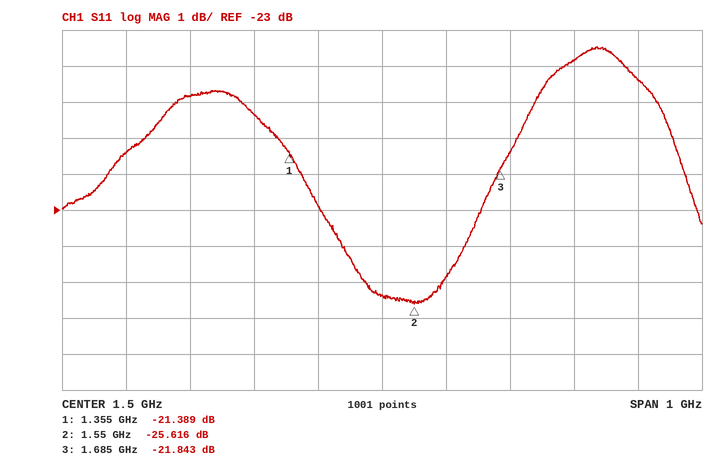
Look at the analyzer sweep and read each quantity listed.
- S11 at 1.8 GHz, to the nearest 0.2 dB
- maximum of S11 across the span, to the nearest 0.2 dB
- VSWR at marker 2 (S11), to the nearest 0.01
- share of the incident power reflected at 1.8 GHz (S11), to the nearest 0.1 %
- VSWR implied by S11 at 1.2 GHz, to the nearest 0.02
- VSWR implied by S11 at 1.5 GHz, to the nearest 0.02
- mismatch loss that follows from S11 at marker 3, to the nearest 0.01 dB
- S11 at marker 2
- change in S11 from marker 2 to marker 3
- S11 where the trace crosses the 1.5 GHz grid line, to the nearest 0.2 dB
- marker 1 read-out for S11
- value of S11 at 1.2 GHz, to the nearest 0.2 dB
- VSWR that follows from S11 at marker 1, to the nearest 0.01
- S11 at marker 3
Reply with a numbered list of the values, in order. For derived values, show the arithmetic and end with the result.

1. -18.8 dB
2. -18.4 dB
3. (1 + 0.0524)/(1 − 0.0524) ≈ 1.11
4. 10^(-18.8/10) ≈ 1.3 %
5. |Γ| = 10^(-19.8/20) = 0.1023; VSWR = (1 + 0.1023)/(1 − 0.1023) ≈ 1.23, so 1.22 to the nearest 0.02
6. |Γ| = 10^(-25.4/20) = 0.0537; VSWR = (1 + 0.0537)/(1 − 0.0537) ≈ 1.11, so 1.12 to the nearest 0.02
7. −10 log10(1 − 10^(-21.843/10)) ≈ 0.03 dB
8. -25.616 dB
9. -21.843 − (-25.616) = 3.773 dB
10. -25.4 dB
11. -21.389 dB
12. -19.8 dB
13. (1 + 0.0852)/(1 − 0.0852) ≈ 1.19
14. -21.843 dB
